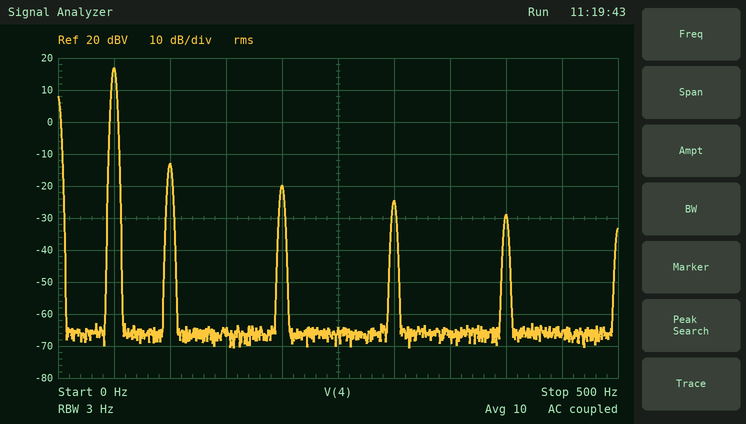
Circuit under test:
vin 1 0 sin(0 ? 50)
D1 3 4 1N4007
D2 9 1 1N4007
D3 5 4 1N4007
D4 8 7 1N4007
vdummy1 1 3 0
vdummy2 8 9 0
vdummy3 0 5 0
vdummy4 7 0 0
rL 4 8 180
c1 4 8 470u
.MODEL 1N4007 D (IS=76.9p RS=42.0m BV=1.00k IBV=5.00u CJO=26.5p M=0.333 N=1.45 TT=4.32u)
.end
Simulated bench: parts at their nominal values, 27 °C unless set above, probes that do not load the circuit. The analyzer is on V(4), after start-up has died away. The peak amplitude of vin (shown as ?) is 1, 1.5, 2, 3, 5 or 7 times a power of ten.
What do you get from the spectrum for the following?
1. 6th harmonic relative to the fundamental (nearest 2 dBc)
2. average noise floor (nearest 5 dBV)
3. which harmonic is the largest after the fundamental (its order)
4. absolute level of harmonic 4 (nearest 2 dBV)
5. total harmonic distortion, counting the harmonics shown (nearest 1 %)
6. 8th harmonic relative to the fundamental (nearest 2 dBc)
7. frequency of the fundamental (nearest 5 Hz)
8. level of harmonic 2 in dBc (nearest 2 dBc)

-42 dBc
-65 dBV
2
-20 dBV
4 %
-46 dBc
50 Hz
-30 dBc
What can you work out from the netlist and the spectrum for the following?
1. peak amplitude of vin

20 V
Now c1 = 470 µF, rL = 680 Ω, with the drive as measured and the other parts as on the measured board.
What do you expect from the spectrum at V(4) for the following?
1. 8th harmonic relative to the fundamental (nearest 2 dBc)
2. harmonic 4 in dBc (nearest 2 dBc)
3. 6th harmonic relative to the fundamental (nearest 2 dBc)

-54 dBc
-48 dBc
-52 dBc
